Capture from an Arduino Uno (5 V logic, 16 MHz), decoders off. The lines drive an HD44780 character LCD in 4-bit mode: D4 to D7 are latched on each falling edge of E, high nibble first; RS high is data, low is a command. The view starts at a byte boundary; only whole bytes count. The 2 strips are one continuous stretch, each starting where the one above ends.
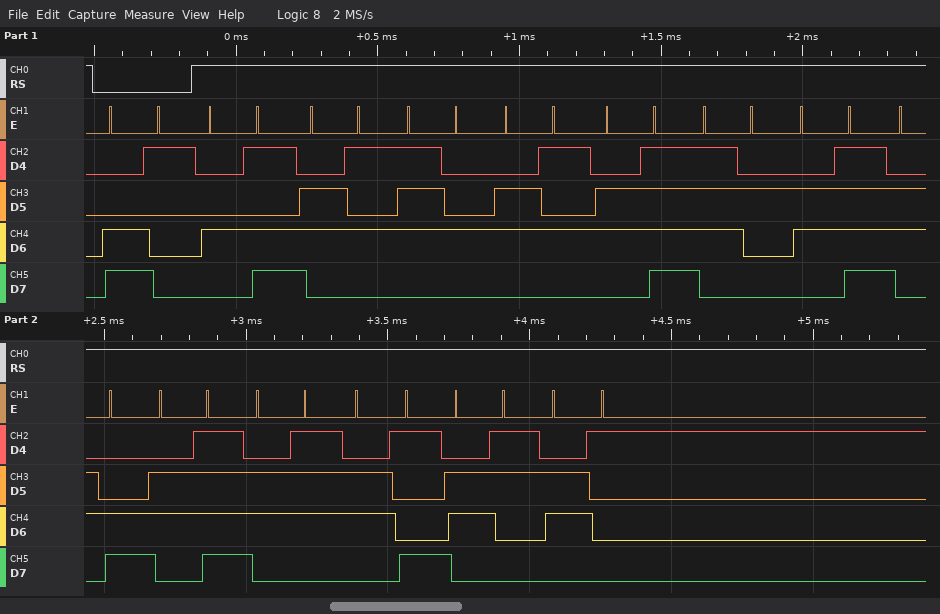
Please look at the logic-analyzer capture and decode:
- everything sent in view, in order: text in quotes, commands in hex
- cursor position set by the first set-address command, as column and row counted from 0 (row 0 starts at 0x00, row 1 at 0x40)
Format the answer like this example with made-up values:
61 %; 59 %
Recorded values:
0xC1 "Meteorologica"; column 1, row 1
